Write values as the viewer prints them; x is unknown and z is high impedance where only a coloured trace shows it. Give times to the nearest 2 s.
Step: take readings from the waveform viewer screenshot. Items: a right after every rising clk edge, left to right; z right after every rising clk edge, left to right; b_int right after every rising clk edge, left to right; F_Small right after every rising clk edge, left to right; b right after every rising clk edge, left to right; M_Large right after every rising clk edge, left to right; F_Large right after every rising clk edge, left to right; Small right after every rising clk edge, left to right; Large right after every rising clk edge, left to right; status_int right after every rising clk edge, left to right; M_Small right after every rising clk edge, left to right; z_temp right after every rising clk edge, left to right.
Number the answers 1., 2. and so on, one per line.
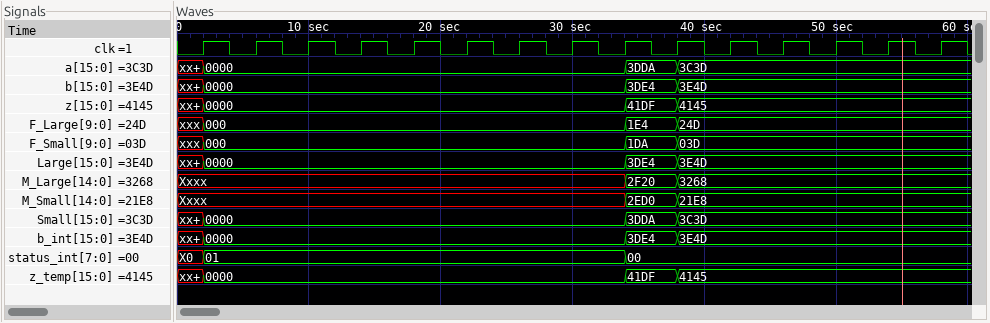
1. 0000, 0000, 0000, 0000, 0000, 0000, 0000, 0000, 3DDA, 3C3D, 3C3D, 3C3D, 3C3D, 3C3D, 3C3D
2. 0000, 0000, 0000, 0000, 0000, 0000, 0000, 0000, 41DF, 4145, 4145, 4145, 4145, 4145, 4145
3. 0000, 0000, 0000, 0000, 0000, 0000, 0000, 0000, 3DE4, 3E4D, 3E4D, 3E4D, 3E4D, 3E4D, 3E4D
4. 000, 000, 000, 000, 000, 000, 000, 000, 1DA, 03D, 03D, 03D, 03D, 03D, 03D
5. 0000, 0000, 0000, 0000, 0000, 0000, 0000, 0000, 3DE4, 3E4D, 3E4D, 3E4D, 3E4D, 3E4D, 3E4D
6. Xxxx, Xxxx, Xxxx, Xxxx, Xxxx, Xxxx, Xxxx, Xxxx, 2F20, 3268, 3268, 3268, 3268, 3268, 3268
7. 000, 000, 000, 000, 000, 000, 000, 000, 1E4, 24D, 24D, 24D, 24D, 24D, 24D
8. 0000, 0000, 0000, 0000, 0000, 0000, 0000, 0000, 3DDA, 3C3D, 3C3D, 3C3D, 3C3D, 3C3D, 3C3D
9. 0000, 0000, 0000, 0000, 0000, 0000, 0000, 0000, 3DE4, 3E4D, 3E4D, 3E4D, 3E4D, 3E4D, 3E4D
10. 01, 01, 01, 01, 01, 01, 01, 01, 00, 00, 00, 00, 00, 00, 00
11. Xxxx, Xxxx, Xxxx, Xxxx, Xxxx, Xxxx, Xxxx, Xxxx, 2ED0, 21E8, 21E8, 21E8, 21E8, 21E8, 21E8
12. 0000, 0000, 0000, 0000, 0000, 0000, 0000, 0000, 41DF, 4145, 4145, 4145, 4145, 4145, 4145
